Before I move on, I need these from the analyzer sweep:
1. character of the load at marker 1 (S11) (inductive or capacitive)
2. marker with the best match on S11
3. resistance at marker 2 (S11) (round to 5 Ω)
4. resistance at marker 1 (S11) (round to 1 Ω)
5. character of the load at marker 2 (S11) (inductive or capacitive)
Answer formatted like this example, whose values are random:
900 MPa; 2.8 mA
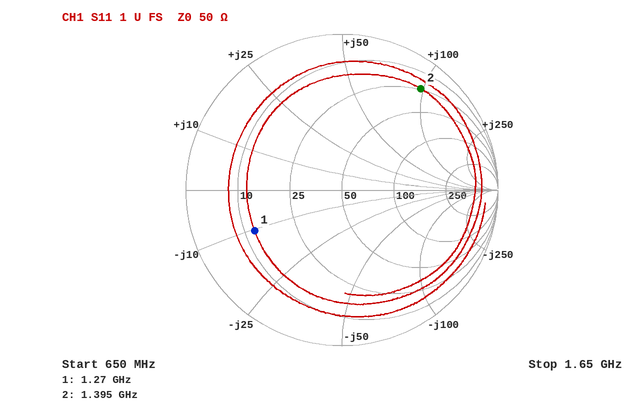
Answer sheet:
capacitive; marker 1; 25 Ω; 12 Ω; inductive
